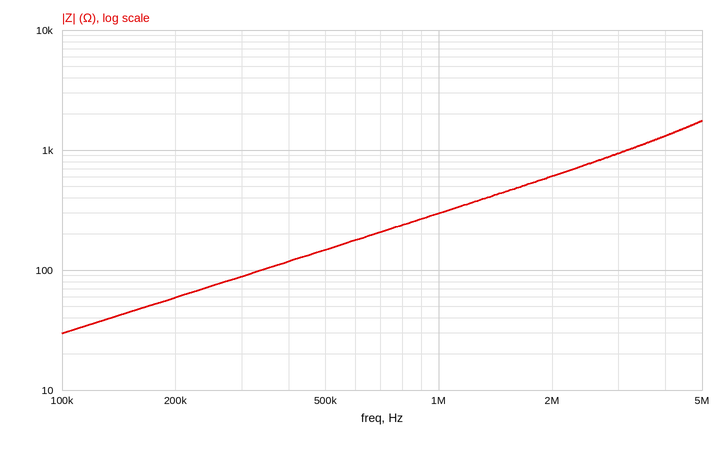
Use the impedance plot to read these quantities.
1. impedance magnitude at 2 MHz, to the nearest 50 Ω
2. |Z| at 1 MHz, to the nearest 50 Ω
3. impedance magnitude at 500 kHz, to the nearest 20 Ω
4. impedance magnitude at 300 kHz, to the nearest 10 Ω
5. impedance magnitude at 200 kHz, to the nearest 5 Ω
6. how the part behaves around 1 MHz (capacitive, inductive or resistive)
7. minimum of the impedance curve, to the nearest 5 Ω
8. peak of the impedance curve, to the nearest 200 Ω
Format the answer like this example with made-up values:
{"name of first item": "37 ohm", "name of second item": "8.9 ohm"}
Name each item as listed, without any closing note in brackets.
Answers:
{"impedance magnitude at 2 MHz, to the nearest 50 Ω": "600 Ω", "|Z| at 1 MHz, to the nearest 50 Ω": "300 Ω", "impedance magnitude at 500 kHz, to the nearest 20 Ω": "140 Ω", "impedance magnitude at 300 kHz, to the nearest 10 Ω": "90 Ω", "impedance magnitude at 200 kHz, to the nearest 5 Ω": "60 Ω", "how the part behaves around 1 MHz": "inductive", "minimum of the impedance curve, to the nearest 5 Ω": "30 Ω", "peak of the impedance curve, to the nearest 200 Ω": "1.8 kΩ"}
